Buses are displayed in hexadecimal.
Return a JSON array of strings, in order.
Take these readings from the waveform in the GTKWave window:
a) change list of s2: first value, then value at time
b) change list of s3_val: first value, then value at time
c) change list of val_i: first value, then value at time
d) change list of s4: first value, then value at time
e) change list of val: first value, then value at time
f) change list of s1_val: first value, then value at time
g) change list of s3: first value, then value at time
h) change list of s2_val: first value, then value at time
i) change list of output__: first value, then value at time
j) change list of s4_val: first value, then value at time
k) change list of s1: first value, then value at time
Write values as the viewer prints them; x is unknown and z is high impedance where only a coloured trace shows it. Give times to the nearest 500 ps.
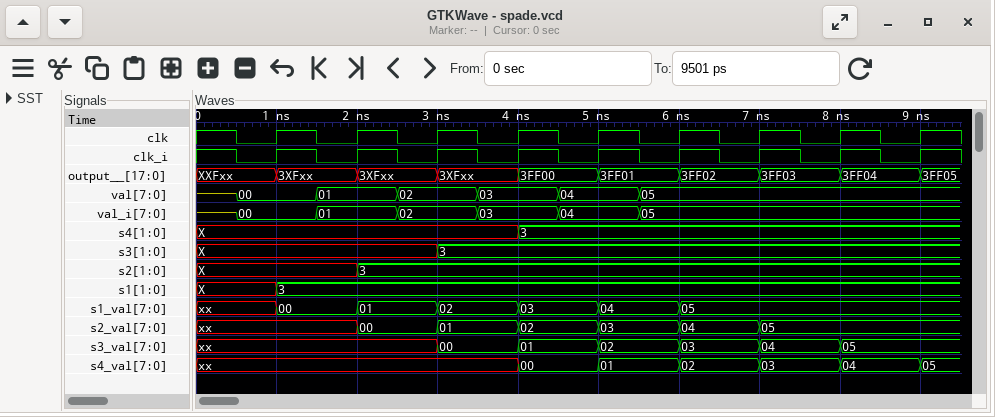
["X, 3 at 2000 ps", "xx, 00 at 3000 ps, 01 at 4000 ps, 02 at 5000 ps, 03 at 6000 ps, 04 at 7000 ps, 05 at 8000 ps", "z, 00 at 500 ps, 01 at 1500 ps, 02 at 2500 ps, 03 at 3500 ps, 04 at 4500 ps, 05 at 5500 ps", "X, 3 at 4000 ps", "z, 00 at 500 ps, 01 at 1500 ps, 02 at 2500 ps, 03 at 3500 ps, 04 at 4500 ps, 05 at 5500 ps", "xx, 00 at 1000 ps, 01 at 2000 ps, 02 at 3000 ps, 03 at 4000 ps, 04 at 5000 ps, 05 at 6000 ps", "X, 3 at 3000 ps", "xx, 00 at 2000 ps, 01 at 3000 ps, 02 at 4000 ps, 03 at 5000 ps, 04 at 6000 ps, 05 at 7000 ps", "XXFxx, 3XFxx at 1000 ps, 3XFxx at 2000 ps, 3XFxx at 3000 ps, 3FF00 at 4000 ps, 3FF01 at 5000 ps, 3FF02 at 6000 ps, 3FF03 at 7000 ps, 3FF04 at 8000 ps, 3FF05 at 9000 ps", "xx, 00 at 4000 ps, 01 at 5000 ps, 02 at 6000 ps, 03 at 7000 ps, 04 at 8000 ps, 05 at 9000 ps", "X, 3 at 1000 ps"]
